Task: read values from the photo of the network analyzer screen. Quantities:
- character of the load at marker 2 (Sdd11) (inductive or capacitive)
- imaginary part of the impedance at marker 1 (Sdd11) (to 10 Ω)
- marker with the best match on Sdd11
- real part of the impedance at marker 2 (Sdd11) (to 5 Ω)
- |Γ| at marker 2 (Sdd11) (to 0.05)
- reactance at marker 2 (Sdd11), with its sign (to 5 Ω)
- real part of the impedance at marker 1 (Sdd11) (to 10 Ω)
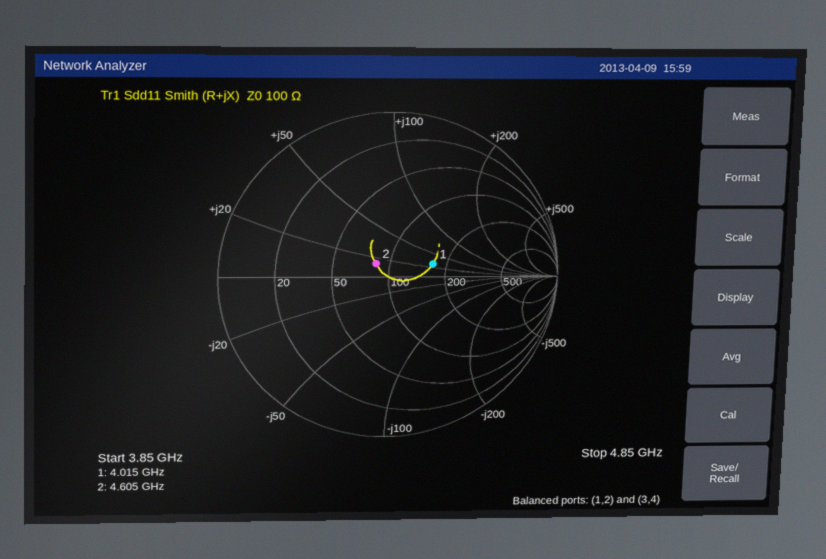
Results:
inductive
+30 Ω
marker 2
85 Ω
0.10
+15 Ω
170 Ω
